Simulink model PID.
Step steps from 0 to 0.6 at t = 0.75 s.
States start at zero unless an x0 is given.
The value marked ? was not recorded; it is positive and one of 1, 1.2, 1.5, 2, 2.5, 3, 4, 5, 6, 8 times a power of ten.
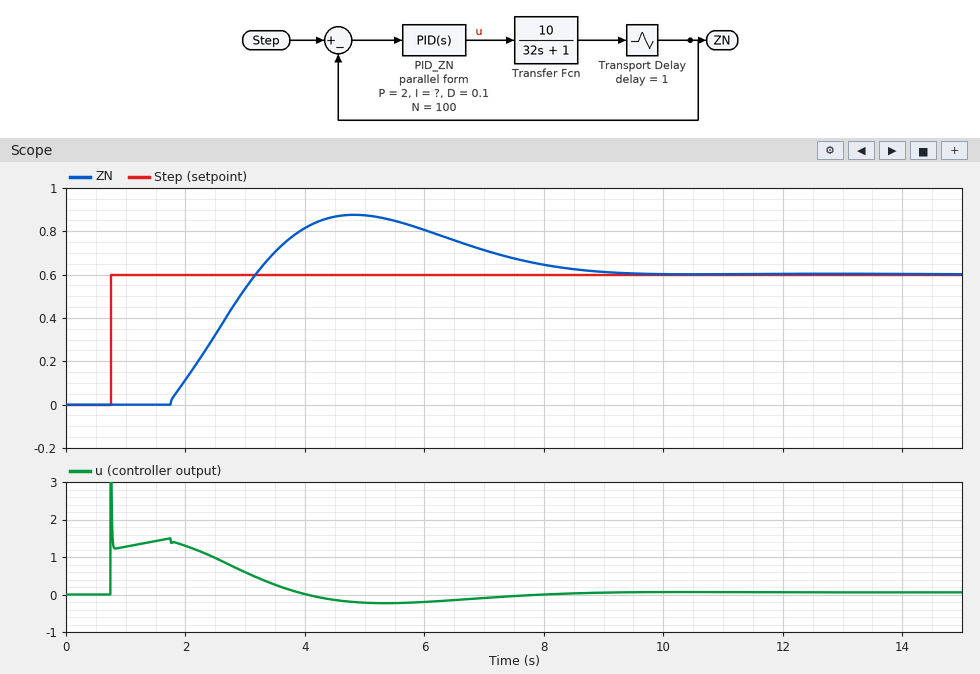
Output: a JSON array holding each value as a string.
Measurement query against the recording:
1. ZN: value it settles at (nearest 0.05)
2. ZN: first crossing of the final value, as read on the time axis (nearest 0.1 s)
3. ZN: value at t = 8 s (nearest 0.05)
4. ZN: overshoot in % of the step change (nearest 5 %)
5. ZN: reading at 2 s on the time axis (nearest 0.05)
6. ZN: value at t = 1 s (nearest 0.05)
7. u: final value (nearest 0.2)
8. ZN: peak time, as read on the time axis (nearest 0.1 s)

["0.60", "3.2 s", "0.65", "45 %", "0.10", "0.00", "0.0", "4.8 s"]
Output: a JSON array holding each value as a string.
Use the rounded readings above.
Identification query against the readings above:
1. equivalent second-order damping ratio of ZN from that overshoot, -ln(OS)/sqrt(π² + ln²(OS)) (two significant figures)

["0.25"]
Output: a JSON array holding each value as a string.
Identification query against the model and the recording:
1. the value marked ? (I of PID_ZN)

["0.5"]
